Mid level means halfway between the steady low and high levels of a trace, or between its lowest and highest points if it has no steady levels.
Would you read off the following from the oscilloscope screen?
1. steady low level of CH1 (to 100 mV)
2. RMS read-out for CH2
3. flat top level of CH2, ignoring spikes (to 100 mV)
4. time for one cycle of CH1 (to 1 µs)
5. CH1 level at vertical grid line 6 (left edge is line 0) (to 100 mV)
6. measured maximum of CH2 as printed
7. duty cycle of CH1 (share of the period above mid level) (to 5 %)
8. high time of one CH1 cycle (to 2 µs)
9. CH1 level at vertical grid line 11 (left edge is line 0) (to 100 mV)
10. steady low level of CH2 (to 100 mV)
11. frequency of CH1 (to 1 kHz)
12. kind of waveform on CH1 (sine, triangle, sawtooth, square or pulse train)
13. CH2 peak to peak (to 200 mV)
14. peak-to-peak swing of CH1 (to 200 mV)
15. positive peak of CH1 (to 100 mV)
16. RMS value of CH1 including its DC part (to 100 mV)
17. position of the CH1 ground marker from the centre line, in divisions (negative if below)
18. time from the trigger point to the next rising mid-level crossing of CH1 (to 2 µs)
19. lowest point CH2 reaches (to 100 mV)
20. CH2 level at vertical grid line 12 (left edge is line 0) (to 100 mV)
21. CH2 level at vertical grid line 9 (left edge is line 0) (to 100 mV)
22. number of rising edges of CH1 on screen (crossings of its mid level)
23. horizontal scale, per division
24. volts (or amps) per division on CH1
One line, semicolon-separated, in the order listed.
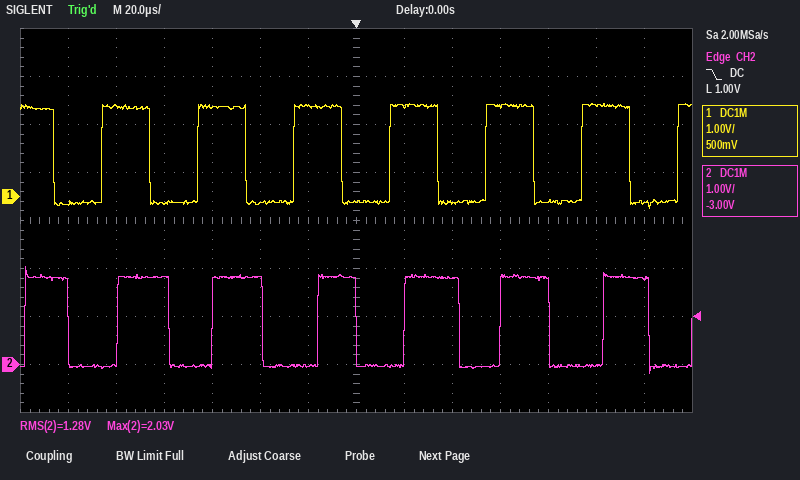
-100 mV; 1.28 V; 1.8 V; 40 µs; 1.9 V; 2.03 V; 50 %; 20 µs; -100 mV; 0.0 V; 25 kHz; square; 2.2 V; 2.2 V; 1.9 V; 1.3 V; +0.5 div; 14 µs; -200 mV; 0.0 V; 1.8 V; 7; 20 µs; 1 V
